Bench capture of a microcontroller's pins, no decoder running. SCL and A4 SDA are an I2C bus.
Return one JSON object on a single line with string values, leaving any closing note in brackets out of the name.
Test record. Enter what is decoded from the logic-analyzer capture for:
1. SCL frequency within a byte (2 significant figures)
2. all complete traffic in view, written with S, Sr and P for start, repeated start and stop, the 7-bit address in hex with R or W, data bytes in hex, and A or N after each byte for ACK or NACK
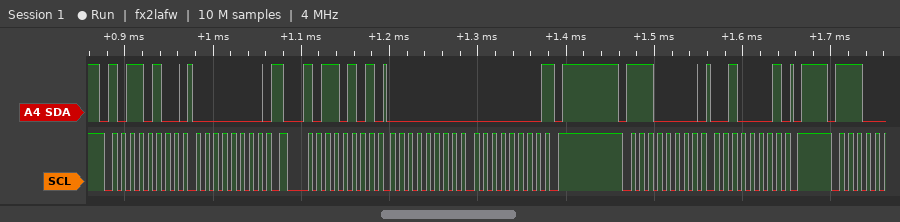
{"SCL frequency within a byte": "100 kHz", "all complete traffic in view, written with S, Sr and P for start, repeated start and stop, the 7-bit address in hex with R or W, data bytes in hex, and A or N after each byte for ACK or NACK": "S 5AW A 00 A Sr 5AR A 00 A 00 N P S 70W A 21 A P"}
